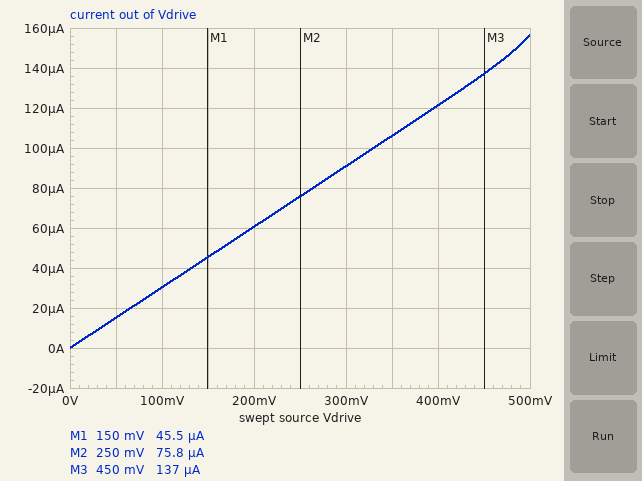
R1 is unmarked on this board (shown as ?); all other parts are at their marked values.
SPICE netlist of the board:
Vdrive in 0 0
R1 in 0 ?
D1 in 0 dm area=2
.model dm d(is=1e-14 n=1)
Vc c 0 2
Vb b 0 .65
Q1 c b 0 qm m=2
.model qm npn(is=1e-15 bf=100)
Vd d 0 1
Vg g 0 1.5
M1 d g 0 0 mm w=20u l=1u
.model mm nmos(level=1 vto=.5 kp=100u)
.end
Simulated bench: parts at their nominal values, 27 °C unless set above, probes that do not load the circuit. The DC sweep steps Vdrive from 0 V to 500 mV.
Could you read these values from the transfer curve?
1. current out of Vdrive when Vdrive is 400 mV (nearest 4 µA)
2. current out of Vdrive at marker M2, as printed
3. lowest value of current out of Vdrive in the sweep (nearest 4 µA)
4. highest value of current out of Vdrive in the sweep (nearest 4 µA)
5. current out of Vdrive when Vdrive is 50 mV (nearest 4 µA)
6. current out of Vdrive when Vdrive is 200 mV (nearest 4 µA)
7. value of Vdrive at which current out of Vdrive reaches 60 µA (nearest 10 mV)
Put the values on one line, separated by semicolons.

120 µA; 75.8 µA; 0 A; 156 µA; 16 µA; 60 µA; 200 mV
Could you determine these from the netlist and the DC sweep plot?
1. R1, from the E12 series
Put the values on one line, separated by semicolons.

3.3 kΩ
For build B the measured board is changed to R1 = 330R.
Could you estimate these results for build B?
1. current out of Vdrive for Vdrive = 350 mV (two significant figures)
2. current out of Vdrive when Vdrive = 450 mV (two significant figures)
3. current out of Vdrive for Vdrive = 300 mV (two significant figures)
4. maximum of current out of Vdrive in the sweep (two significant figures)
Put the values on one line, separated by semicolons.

1.1 mA; 1.4 mA; 910 µA; 1.5 mA
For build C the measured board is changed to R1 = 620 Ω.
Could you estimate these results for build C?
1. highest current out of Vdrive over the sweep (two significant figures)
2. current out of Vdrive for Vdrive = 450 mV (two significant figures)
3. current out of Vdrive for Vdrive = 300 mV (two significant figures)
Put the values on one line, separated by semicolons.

810 µA; 730 µA; 480 µA
